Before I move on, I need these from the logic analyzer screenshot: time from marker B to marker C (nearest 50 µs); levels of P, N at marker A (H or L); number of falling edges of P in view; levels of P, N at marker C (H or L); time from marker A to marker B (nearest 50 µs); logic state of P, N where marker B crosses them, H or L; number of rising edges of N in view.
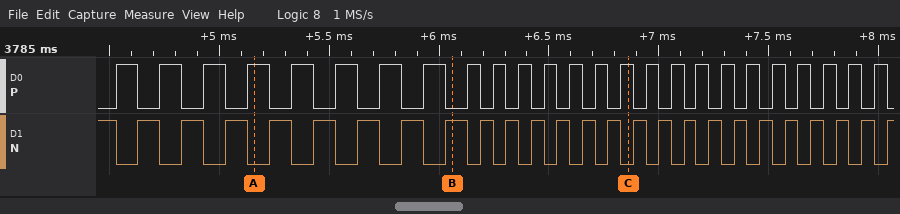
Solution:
800 µs
P=H, N=L
25
P=H, N=L
900 µs
P=L, N=H
25
